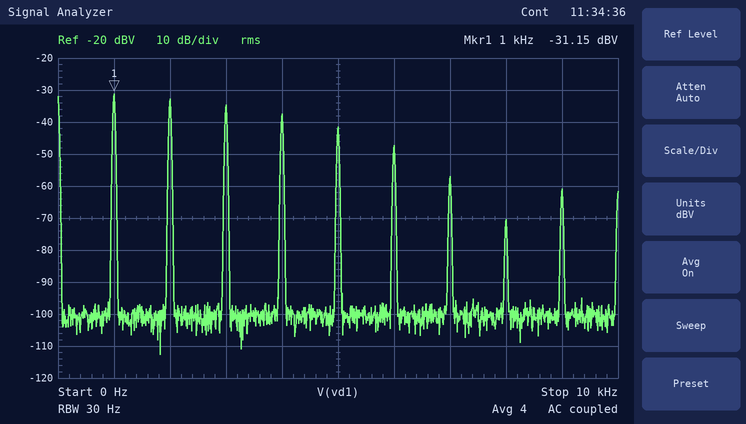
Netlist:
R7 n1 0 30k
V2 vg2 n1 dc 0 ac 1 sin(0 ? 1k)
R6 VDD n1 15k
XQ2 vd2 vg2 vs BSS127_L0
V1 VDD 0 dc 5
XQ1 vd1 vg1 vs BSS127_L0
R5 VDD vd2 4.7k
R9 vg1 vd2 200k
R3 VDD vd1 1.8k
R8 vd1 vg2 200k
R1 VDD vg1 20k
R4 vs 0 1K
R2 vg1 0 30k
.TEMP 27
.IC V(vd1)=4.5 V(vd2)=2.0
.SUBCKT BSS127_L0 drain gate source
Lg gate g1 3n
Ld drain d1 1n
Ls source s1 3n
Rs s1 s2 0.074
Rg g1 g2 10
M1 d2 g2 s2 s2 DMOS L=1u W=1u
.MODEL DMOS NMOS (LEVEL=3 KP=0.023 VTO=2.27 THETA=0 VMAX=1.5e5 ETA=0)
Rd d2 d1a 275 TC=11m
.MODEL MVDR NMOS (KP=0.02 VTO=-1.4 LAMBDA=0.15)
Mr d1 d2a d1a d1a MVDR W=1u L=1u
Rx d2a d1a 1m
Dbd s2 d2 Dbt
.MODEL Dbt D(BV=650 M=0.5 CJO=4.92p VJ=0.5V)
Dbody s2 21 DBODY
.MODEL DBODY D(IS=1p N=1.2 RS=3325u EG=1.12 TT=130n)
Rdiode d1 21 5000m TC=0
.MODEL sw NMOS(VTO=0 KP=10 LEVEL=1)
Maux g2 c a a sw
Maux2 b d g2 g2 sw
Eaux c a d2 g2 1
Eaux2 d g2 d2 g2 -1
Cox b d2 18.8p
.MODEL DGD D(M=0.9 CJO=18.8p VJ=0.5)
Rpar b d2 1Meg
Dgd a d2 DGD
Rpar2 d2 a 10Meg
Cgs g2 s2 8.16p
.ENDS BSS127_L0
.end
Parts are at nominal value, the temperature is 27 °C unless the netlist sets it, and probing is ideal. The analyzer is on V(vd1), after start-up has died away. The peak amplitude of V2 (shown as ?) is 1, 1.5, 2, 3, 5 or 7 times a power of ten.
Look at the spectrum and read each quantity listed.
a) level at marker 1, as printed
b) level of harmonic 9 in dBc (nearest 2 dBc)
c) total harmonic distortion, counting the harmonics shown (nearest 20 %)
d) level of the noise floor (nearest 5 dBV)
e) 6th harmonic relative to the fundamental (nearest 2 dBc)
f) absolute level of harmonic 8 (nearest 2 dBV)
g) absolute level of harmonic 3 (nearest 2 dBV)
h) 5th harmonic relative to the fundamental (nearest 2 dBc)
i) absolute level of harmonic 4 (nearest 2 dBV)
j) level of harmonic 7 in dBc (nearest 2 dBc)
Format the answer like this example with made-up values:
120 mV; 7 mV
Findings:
-31.15 dBV; -30 dBc; 120 %; -100 dBV; -16 dBc; -70 dBV; -34 dBV; -10 dBc; -38 dBV; -26 dBc
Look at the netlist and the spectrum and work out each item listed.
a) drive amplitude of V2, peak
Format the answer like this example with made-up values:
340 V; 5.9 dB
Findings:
300 mV
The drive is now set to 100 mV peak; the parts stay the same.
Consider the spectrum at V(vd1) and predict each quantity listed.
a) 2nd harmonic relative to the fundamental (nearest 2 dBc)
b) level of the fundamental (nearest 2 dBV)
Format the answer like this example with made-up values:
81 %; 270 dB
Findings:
-44 dBc; -64 dBV
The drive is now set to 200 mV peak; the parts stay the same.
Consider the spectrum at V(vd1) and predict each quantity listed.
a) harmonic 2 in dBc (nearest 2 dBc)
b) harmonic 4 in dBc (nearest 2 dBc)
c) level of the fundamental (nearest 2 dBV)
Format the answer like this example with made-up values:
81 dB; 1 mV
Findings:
-42 dBc; -58 dBc; -58 dBV
